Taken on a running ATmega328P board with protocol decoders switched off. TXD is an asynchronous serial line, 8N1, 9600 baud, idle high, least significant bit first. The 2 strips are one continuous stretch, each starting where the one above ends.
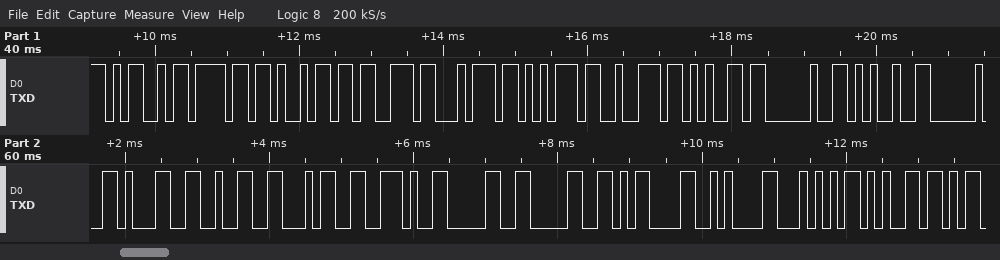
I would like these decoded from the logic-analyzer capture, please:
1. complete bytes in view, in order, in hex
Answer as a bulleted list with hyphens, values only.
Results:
- 4D 6F 69 73 74 75 72 65 20 25 20 31 32 34 2E 30 30 0D 0A 54 65
